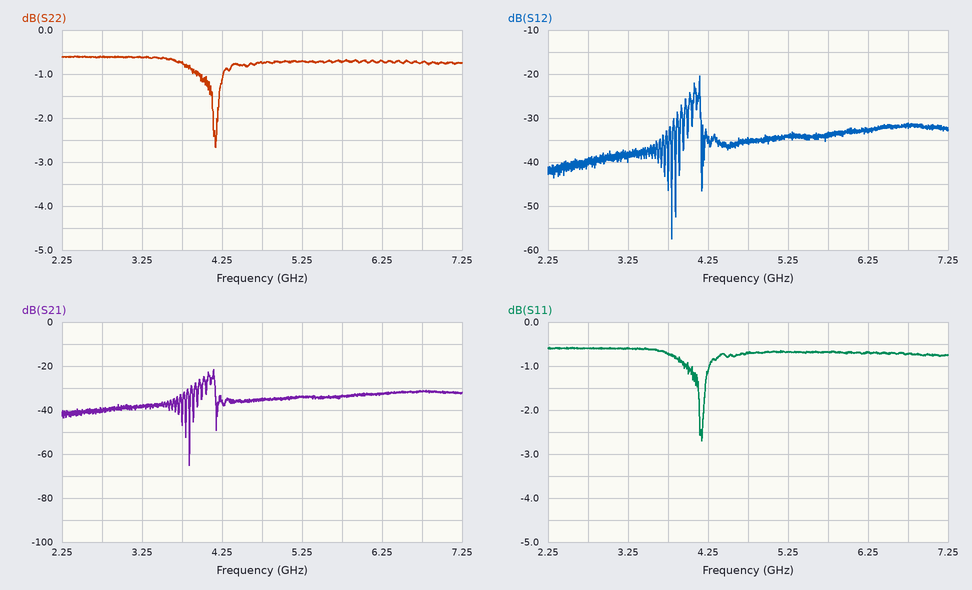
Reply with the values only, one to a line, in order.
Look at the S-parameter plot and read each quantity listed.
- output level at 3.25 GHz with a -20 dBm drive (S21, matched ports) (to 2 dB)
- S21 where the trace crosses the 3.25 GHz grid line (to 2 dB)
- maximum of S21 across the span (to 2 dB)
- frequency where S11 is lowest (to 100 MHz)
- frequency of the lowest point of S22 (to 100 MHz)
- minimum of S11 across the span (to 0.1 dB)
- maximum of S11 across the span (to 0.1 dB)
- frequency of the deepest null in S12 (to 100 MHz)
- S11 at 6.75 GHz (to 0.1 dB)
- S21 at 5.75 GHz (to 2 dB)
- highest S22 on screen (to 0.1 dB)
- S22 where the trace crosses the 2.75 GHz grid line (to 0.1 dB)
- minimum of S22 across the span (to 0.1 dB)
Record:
-58 dBm
-38 dB
-22 dB
4.2 GHz
4.2 GHz
-2.7 dB
-0.6 dB
3.8 GHz
-0.7 dB
-34 dB
-0.6 dB
-0.6 dB
-2.7 dB
